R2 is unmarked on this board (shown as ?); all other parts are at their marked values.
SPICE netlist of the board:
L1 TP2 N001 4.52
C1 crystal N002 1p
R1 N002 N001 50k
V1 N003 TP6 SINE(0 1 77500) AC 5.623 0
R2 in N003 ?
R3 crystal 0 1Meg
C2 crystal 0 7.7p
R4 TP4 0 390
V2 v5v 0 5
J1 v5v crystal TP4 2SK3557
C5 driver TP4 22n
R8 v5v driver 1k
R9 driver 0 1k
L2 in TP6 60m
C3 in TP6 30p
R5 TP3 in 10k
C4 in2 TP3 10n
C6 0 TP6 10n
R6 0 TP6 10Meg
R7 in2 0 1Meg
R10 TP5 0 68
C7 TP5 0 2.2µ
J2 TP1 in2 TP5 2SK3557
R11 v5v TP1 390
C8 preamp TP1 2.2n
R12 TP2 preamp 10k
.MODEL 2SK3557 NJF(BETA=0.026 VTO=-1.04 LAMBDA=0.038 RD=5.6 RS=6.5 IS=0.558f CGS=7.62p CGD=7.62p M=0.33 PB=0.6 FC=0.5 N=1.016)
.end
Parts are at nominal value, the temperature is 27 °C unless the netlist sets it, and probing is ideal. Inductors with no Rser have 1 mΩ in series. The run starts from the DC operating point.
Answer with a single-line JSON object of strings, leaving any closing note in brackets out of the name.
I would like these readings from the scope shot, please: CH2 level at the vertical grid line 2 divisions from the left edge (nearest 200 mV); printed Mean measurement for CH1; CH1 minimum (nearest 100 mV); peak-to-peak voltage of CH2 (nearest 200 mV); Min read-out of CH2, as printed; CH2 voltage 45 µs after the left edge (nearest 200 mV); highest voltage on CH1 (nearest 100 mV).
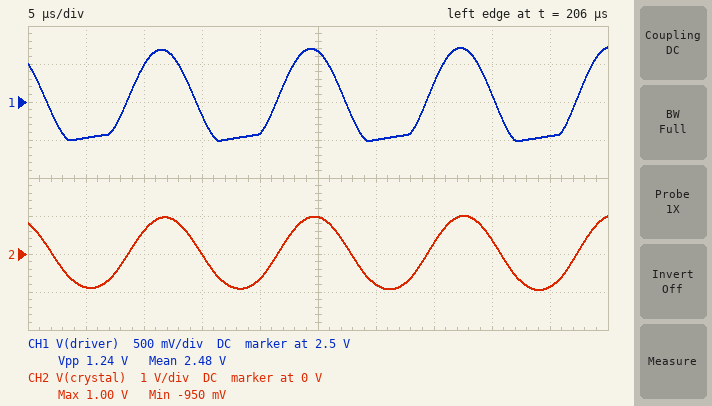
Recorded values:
{"CH2 level at the vertical grid line 2 divisions from the left edge": "600 mV", "printed Mean measurement for CH1": "2.48 V", "CH1 minimum": "2.0 V", "peak-to-peak voltage of CH2": "2.0 V", "Min read-out of CH2, as printed": "-950 mV", "CH2 voltage 45 µs after the left edge": "-800 mV", "highest voltage on CH1": "3.2 V"}
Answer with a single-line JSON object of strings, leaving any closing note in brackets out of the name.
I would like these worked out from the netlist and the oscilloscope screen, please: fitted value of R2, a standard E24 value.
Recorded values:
{"fitted value of R2, a standard E24 value": "3 MΩ"}
